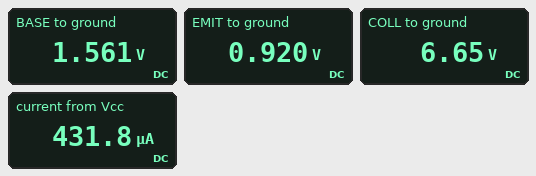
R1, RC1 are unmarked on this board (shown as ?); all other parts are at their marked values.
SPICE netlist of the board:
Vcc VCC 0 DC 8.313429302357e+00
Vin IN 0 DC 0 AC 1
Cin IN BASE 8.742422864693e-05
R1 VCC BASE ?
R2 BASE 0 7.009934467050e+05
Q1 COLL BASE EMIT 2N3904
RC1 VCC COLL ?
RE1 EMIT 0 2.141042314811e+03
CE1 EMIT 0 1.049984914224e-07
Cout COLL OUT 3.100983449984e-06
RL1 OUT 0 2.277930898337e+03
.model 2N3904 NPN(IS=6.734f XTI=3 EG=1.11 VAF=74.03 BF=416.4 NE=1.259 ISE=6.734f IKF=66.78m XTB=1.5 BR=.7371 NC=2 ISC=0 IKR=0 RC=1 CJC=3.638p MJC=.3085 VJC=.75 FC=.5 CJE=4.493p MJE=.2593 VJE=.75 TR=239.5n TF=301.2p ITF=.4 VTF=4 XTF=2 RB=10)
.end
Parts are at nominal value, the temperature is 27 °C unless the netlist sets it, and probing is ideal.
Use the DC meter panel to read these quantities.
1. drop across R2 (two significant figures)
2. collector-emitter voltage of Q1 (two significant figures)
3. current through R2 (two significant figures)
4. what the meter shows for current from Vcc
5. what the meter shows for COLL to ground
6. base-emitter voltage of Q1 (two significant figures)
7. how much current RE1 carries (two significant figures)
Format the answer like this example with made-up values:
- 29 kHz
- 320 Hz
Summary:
- 1.6 V
- 5.7 V
- 2.2 µA
- 431.8 µA
- 6.65 V
- 640 mV
- 430 µA
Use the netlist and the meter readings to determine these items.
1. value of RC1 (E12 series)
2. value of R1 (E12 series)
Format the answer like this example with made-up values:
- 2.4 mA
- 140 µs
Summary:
- 3.9 kΩ
- 1.2 MΩ
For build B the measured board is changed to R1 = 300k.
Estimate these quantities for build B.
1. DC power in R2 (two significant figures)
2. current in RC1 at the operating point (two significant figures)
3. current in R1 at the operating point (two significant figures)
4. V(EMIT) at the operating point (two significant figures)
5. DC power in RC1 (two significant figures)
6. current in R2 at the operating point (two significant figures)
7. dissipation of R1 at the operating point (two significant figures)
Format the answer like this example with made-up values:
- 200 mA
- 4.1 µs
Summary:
- 18 µW
- 1.3 mA
- 16 µA
- 2.9 V
- 7.0 mW
- 5.1 µA
- 75 µW
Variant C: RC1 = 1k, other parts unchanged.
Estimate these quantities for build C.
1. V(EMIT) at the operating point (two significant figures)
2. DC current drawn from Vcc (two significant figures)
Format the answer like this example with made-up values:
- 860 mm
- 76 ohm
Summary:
- 930 mV
- 440 µA
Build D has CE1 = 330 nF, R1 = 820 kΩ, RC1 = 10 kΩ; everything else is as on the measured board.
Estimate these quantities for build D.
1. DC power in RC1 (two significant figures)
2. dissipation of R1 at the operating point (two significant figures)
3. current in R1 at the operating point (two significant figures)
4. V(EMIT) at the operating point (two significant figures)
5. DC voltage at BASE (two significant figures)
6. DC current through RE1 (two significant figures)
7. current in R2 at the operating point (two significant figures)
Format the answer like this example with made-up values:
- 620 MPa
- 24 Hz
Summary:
- 3.8 mW
- 49 µW
- 7.7 µA
- 1.3 V
- 2.0 V
- 620 µA
- 2.8 µA
